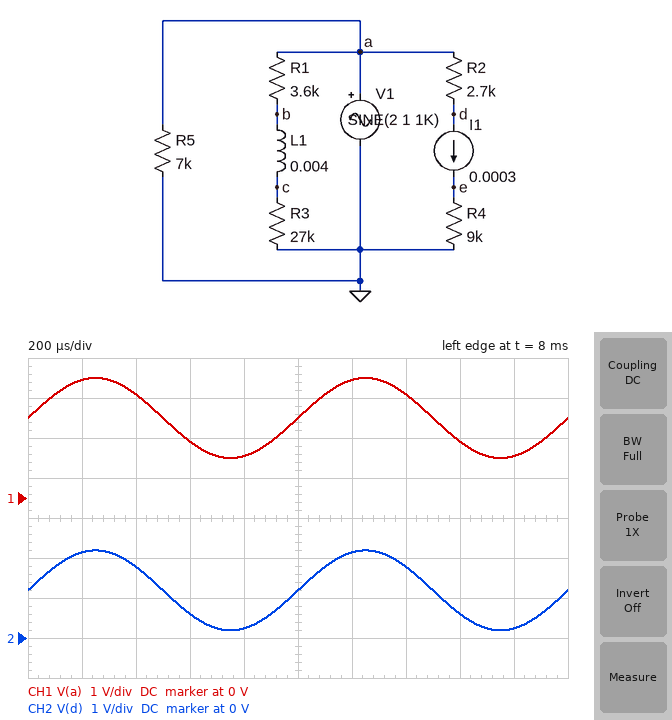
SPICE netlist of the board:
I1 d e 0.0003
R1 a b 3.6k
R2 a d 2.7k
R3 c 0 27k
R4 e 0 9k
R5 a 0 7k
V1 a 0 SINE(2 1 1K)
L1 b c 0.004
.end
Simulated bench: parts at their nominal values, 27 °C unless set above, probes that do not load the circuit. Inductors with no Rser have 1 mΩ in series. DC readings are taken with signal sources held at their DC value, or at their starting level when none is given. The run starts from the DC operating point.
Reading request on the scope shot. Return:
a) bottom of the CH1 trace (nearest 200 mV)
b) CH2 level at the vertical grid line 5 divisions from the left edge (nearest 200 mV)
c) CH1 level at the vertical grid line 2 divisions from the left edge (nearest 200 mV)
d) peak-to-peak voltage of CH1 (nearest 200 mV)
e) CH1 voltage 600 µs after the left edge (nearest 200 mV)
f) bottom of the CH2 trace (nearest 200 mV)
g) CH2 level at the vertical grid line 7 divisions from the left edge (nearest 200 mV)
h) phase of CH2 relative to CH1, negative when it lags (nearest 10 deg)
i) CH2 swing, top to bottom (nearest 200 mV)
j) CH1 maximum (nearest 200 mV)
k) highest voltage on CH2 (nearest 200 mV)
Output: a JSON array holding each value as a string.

["1.0 V", "1.2 V", "2.6 V", "2.0 V", "1.4 V", "200 mV", "1.8 V", "0 deg", "2.0 V", "3.0 V", "2.2 V"]
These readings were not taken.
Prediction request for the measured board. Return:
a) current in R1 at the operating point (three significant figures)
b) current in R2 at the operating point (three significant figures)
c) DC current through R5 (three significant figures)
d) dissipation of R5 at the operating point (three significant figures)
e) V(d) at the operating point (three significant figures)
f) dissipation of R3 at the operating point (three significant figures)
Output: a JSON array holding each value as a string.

["65.4 µA", "300 µA", "286 µA", "571 µW", "1.19 V", "115 µW"]
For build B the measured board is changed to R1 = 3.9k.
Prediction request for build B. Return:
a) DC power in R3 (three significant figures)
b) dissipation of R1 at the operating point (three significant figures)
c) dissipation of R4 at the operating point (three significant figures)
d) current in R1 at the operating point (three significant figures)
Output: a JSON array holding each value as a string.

["113 µW", "16.3 µW", "810 µW", "64.7 µA"]
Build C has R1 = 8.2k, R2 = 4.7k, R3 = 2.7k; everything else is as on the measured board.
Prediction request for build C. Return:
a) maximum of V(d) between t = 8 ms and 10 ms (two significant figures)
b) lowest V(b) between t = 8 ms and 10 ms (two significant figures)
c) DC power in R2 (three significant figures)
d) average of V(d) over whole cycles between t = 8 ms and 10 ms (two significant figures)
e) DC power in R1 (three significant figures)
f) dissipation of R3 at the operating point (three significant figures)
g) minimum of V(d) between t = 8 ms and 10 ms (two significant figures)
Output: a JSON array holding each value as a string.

["1.6 V", "250 mV", "423 µW", "590 mV", "276 µW", "90.9 µW", "-410 mV"]
